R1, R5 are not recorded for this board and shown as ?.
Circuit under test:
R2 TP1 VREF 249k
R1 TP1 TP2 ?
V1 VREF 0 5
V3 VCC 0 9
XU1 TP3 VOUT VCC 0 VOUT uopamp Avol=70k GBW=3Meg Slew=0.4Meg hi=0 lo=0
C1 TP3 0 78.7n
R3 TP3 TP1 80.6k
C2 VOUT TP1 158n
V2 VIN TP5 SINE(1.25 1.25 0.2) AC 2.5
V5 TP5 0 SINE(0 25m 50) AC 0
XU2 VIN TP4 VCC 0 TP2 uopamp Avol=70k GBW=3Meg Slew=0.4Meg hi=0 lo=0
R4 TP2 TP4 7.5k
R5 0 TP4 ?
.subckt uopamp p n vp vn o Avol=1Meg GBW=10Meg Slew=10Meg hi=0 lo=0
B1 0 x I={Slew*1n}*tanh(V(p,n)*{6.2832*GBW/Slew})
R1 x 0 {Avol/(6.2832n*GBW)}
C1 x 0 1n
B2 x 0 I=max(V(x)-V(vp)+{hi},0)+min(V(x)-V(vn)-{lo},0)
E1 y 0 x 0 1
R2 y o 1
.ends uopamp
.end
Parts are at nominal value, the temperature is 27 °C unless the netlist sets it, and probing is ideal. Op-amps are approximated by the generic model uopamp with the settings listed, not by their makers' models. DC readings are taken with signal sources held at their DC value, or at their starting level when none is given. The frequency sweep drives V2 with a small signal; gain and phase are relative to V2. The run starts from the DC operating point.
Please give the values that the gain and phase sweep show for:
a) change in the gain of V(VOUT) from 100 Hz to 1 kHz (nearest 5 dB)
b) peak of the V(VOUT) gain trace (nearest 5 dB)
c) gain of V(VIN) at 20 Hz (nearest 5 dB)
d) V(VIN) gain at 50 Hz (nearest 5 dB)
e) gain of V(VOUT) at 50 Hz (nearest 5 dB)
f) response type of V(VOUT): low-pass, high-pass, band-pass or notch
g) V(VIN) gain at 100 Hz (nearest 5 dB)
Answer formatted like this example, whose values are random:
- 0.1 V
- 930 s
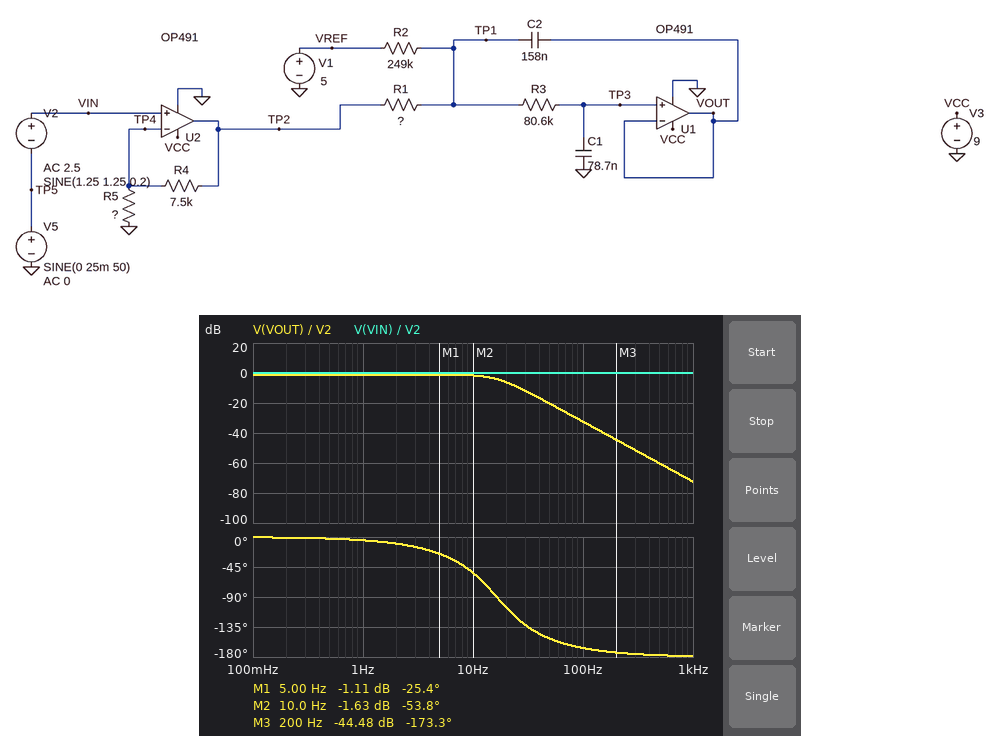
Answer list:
- -40 dB
- 0 dB
- 0 dB
- 0 dB
- -20 dB
- low-pass
- 0 dB
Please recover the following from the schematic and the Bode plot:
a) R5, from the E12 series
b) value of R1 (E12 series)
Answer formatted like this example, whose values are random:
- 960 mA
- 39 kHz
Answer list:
- 18 kΩ
- 150 kΩ
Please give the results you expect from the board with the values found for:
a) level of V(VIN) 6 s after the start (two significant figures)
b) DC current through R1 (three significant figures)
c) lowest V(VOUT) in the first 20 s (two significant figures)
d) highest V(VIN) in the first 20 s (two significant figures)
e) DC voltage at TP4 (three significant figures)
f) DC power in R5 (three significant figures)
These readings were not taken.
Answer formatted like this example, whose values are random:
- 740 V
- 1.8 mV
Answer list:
- 2.4 V
- 8.09 µA
- 1.9 V
- 2.5 V
- 1.25 V
- 86.8 µW
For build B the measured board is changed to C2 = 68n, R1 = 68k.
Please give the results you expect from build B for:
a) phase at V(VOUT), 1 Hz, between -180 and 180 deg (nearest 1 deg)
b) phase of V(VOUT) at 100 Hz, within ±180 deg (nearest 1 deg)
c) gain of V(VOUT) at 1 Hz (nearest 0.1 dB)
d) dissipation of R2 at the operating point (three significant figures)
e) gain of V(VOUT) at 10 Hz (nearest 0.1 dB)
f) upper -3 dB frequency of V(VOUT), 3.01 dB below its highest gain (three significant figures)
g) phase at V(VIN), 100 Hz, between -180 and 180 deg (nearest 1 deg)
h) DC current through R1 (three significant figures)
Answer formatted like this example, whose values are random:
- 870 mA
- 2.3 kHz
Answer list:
- -4 deg
- -141 deg
- 0.9 dB
- 25.8 µW
- -0.1 dB
- 18.7 Hz
- 0 deg
- 10.2 µA
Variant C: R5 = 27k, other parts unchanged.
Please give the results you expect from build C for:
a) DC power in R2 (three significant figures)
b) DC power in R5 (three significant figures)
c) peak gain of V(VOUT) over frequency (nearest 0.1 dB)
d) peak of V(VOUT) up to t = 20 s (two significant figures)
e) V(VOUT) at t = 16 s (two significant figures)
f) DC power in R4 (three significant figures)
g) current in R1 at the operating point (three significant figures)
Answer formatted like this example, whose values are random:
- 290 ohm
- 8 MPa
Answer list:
- 18.1 µW
- 57.9 µW
- -2.0 dB
- 3.9 V
- 3.8 V
- 16.1 µW
- 8.53 µA
